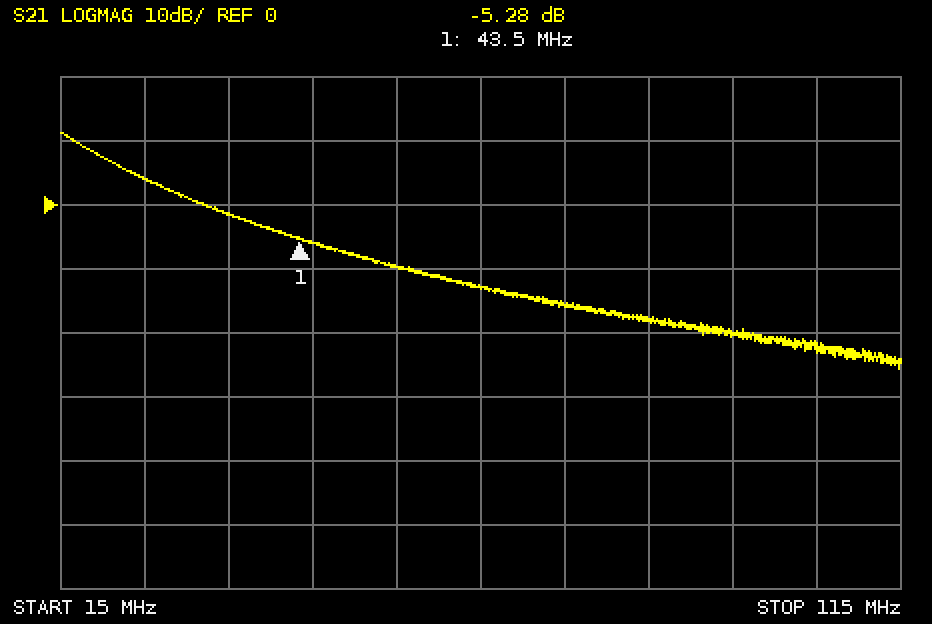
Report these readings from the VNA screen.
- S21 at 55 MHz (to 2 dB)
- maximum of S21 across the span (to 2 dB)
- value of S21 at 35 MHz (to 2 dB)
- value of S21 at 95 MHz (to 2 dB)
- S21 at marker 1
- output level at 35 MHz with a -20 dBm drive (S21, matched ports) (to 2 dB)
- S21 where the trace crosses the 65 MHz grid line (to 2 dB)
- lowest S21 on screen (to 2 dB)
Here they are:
-10 dB
12 dB
-2 dB
-20 dB
-5.28 dB
-22 dBm
-12 dB
-26 dB
